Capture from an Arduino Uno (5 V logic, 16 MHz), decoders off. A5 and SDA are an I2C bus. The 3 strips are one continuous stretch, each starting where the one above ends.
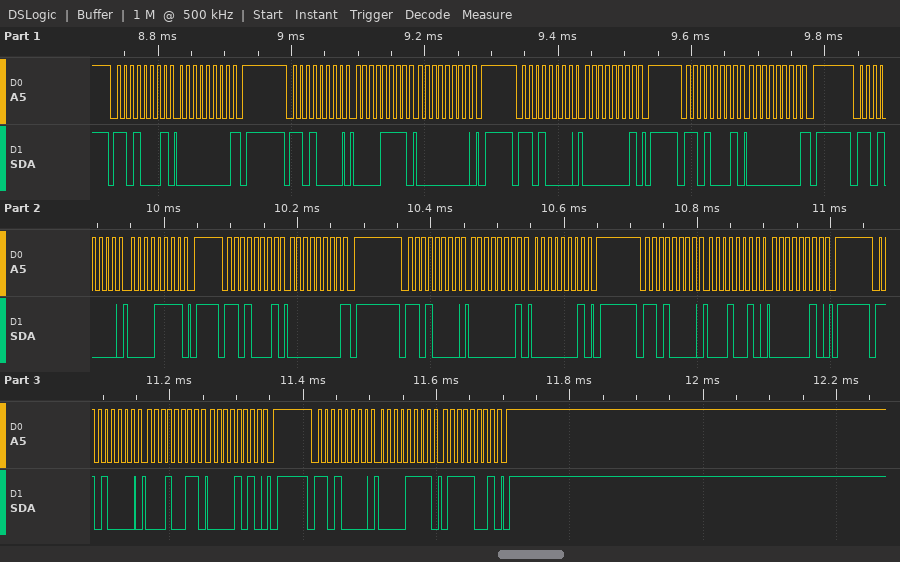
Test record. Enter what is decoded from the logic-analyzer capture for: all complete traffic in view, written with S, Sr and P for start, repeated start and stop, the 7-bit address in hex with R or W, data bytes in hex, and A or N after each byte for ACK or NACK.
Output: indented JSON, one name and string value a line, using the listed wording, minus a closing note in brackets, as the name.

{
  "all complete traffic in view, written with S, Sr and P for start, repeated start and stop, the 7-bit address in hex with R or W, data bytes in hex, and A or N after each byte for ACK or NACK": "S 68R A 00 N P S 68W A 0F A 00 A P S 68W A 01 A P S 68R A 00 N P S 68W A 0F A P S 68R A 00 N P S 68W A 01 A 01 A P S 68W A 12 A 02 A P S 68W A 13 A 0A A P S 68W A 0F A 79 A P"
}
